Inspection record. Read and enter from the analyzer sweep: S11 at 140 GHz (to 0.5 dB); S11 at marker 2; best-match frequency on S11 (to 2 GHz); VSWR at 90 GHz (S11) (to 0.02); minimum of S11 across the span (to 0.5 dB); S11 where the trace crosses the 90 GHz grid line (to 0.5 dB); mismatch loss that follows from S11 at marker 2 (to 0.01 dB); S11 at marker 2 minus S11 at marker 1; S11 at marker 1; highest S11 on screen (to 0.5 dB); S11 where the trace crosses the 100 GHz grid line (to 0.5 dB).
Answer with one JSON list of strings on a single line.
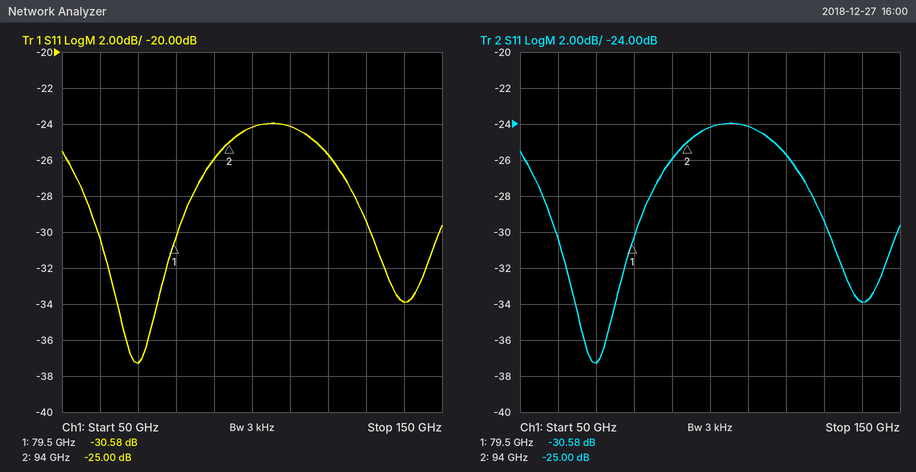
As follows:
["-34.0 dB", "-25.00 dB", "70 GHz", "1.10", "-37.5 dB", "-26.0 dB", "0.01 dB", "5.58 dB", "-30.58 dB", "-24.0 dB", "-24.0 dB"]
